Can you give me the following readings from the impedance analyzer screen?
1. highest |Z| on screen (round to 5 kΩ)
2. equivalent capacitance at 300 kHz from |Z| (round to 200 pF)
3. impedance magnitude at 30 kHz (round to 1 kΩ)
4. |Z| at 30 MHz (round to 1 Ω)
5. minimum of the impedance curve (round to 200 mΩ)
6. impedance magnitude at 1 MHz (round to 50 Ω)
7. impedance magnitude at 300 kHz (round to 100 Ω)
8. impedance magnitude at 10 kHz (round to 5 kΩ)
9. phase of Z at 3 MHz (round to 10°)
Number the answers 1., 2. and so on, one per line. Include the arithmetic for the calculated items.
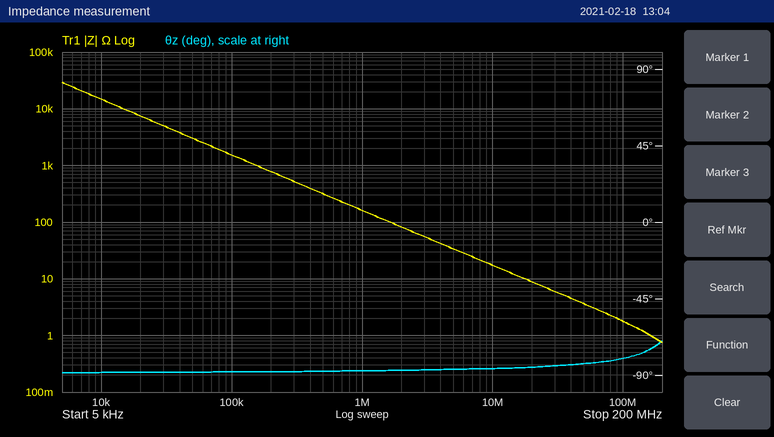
1. 30 kΩ
2. C = 1/(2π × 300 kHz × 500 Ω) ≈ 1.06 nF, so 1.0 nF to the nearest 200 pF
3. 5 kΩ
4. 6 Ω
5. 800 mΩ
6. 150 Ω
7. 500 Ω
8. 15 kΩ
9. -90°
